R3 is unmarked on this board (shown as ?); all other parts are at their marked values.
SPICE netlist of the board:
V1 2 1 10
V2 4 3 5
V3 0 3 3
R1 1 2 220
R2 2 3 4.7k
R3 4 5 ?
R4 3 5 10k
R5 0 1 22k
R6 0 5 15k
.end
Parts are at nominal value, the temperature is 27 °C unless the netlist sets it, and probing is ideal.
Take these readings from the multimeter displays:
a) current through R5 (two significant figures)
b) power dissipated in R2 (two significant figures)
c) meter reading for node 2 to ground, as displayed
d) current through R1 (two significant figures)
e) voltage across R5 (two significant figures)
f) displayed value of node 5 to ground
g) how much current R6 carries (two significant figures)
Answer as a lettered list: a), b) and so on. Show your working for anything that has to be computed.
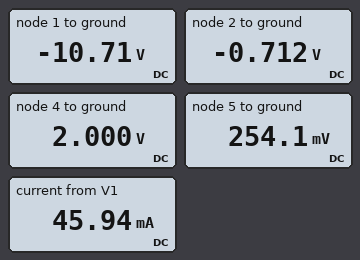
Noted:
a) (0 V - (-10.71 V)) / 22 kΩ = 490 µA
b) (-712 mV - (-3 V))^2 / 4.7 kΩ = 1.1 mW
c) -0.712 V
d) (-712 mV - (-10.71 V)) / 220 Ω = 45 mA
e) 0 V - (-10.71 V) = 11 V
f) 254.1 mV
g) (254.1 mV) / 15 kΩ = 17 µA
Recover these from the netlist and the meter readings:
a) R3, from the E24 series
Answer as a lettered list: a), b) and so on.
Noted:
a) 5.1 kΩ
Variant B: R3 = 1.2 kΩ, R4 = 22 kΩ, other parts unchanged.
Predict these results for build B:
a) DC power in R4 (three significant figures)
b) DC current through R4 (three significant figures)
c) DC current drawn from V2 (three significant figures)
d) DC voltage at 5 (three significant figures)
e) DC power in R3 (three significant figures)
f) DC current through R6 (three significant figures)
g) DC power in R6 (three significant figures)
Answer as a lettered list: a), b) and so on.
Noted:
a) 970 µW
b) 210 µA
c) 318 µA
d) 1.62 V
e) 121 µW
f) 108 µA
g) 175 µW
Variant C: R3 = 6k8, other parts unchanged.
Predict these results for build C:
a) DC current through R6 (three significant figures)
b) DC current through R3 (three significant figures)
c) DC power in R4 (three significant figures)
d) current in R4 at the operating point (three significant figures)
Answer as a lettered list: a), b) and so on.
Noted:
a) 1.25 µA
b) 297 µA
c) 889 µW
d) 298 µA
